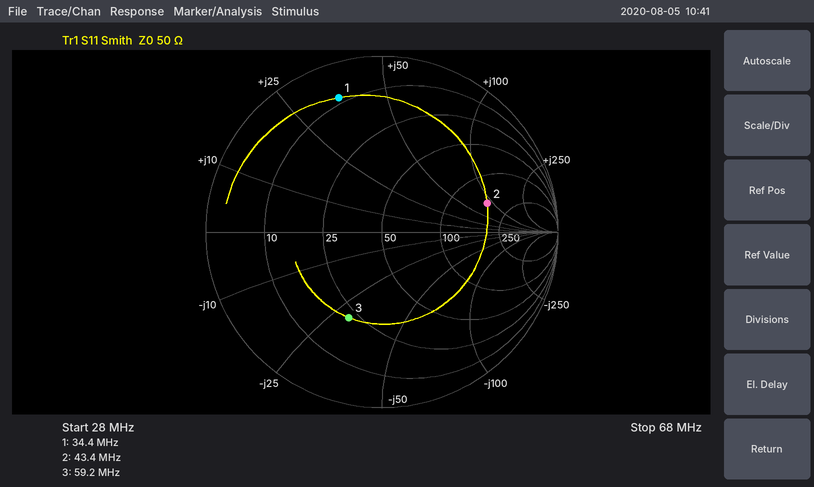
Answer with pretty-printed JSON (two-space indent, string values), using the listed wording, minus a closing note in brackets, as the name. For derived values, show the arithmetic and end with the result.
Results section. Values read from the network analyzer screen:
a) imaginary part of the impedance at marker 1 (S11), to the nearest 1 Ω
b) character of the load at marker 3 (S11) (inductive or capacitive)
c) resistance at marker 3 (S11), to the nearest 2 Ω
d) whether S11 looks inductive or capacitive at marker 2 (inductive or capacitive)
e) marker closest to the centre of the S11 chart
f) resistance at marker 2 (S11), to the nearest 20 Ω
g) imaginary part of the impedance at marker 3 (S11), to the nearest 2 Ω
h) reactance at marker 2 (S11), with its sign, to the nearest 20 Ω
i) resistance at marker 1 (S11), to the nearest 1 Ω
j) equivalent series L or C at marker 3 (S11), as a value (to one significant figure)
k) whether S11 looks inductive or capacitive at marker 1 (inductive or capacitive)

{
  "imaginary part of the impedance at marker 1 (S11), to the nearest 1 Ω": "+36 Ω",
  "character of the load at marker 3 (S11)": "capacitive",
  "resistance at marker 3 (S11), to the nearest 2 Ω": "22 Ω",
  "whether S11 looks inductive or capacitive at marker 2": "inductive",
  "marker closest to the centre of the S11 chart": "marker 3",
  "resistance at marker 2 (S11), to the nearest 20 Ω": "160 Ω",
  "imaginary part of the impedance at marker 3 (S11), to the nearest 2 Ω": "-30 Ω",
  "reactance at marker 2 (S11), with its sign, to the nearest 20 Ω": "+80 Ω",
  "resistance at marker 1 (S11), to the nearest 1 Ω": "8 Ω",
  "equivalent series L or C at marker 3 (S11), as a value": "C = 1/(2π × 59.2 MHz × 30 Ω) ≈ 90 pF",
  "whether S11 looks inductive or capacitive at marker 1": "inductive"
}
